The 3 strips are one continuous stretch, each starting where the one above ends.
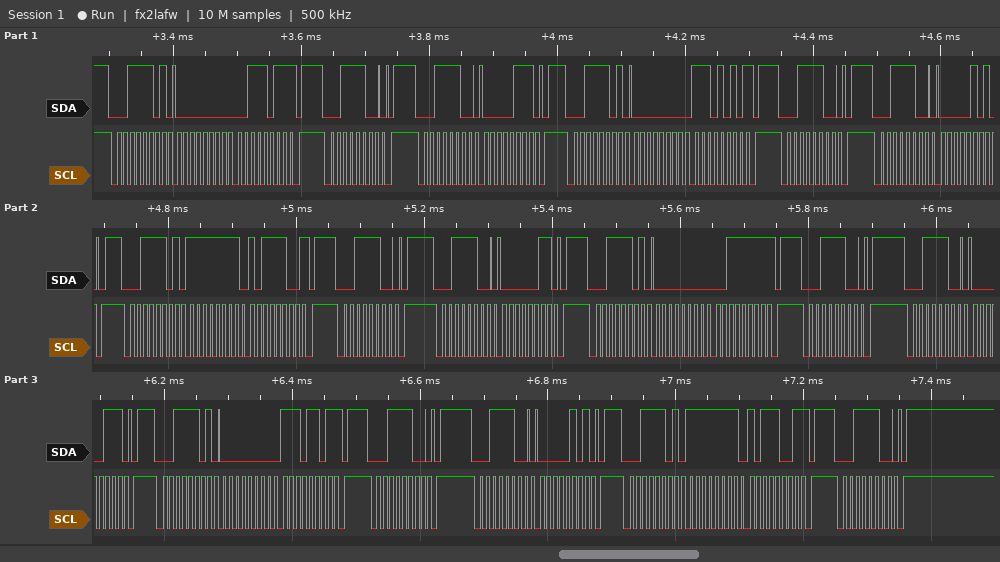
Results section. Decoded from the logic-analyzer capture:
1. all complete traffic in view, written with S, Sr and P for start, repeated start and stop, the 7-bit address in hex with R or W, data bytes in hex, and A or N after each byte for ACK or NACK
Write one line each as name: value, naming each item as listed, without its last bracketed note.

all complete traffic in view, written with S, Sr and P for start, repeated start and stop, the 7-bit address in hex with R or W, data bytes in hex, and A or N after each byte for ACK or NACK: S 1ER A 00 A 3B N P S 1EW A P S 1EW A 07 A P S 1ER A 00 A EA N P S 1EW A P S 1EW A 05 A P S 1ER A FF A BC N P S 1EW A P S 1EW A 03 A P S 1ER A 00 A 3F N P S 1EW A P S 1EW A 07 A P S 1ER A 00 A ED N P S 1EW A P S 1EW A 05 A P S 1ER A FF A B9 N P S 1EW A P
